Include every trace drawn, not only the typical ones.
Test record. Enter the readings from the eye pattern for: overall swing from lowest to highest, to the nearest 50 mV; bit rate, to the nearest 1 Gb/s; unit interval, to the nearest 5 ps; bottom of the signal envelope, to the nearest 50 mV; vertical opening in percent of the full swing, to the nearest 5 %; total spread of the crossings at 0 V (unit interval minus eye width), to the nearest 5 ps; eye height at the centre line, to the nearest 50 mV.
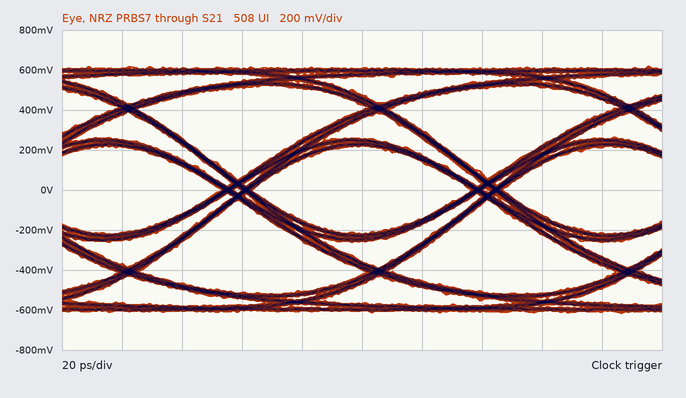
1.25 V
12 Gb/s
85 ps
-600 mV
35 %
10 ps
450 mV
